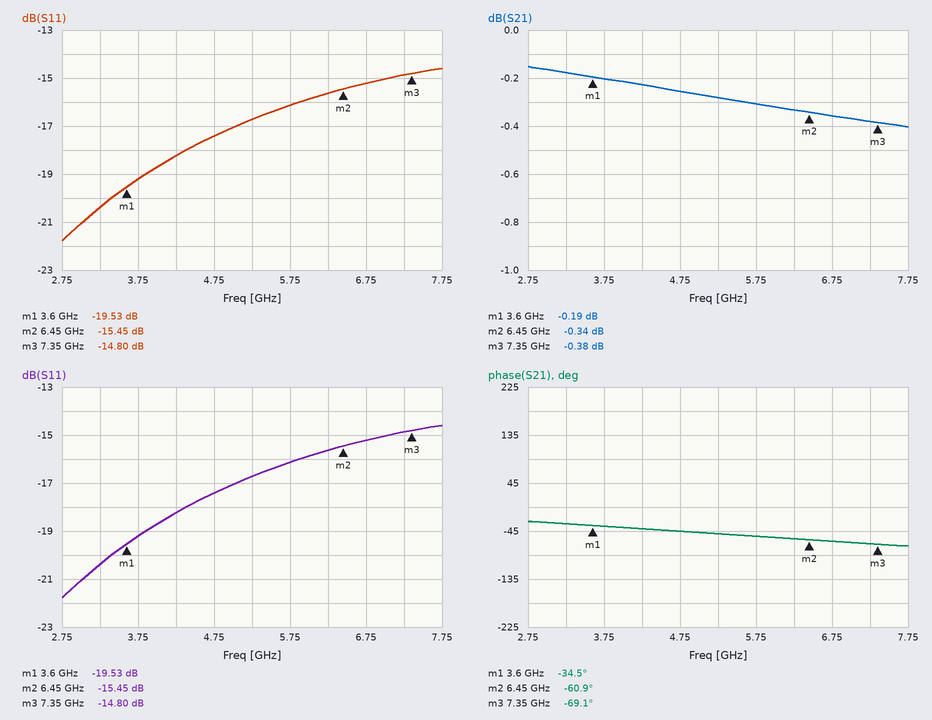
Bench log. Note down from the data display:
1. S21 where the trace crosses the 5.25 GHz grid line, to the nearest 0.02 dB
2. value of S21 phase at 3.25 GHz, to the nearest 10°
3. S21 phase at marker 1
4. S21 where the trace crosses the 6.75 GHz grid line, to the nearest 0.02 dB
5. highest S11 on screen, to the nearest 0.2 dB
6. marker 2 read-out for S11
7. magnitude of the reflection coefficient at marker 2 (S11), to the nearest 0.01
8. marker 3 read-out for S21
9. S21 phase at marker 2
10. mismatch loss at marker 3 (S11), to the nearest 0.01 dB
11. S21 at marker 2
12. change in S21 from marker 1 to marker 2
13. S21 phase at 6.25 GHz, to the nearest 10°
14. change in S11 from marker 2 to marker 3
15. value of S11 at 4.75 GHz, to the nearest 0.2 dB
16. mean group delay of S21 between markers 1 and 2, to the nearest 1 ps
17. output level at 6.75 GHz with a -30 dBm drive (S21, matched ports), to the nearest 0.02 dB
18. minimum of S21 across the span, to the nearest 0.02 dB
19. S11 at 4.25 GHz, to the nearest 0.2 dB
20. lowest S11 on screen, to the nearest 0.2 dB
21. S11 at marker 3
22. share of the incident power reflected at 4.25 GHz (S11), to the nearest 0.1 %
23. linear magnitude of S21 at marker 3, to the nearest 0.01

-0.28 dB
-30°
-34.5°
-0.36 dB
-14.6 dB
-15.45 dB
0.17
-0.38 dB
-60.9°
0.15 dB
-0.34 dB
-0.15 dB
-60°
0.65 dB
-17.4 dB
26 ps
-30.36 dBm
-0.40 dB
-18.2 dB
-21.8 dB
-14.80 dB
1.5 %
0.96
